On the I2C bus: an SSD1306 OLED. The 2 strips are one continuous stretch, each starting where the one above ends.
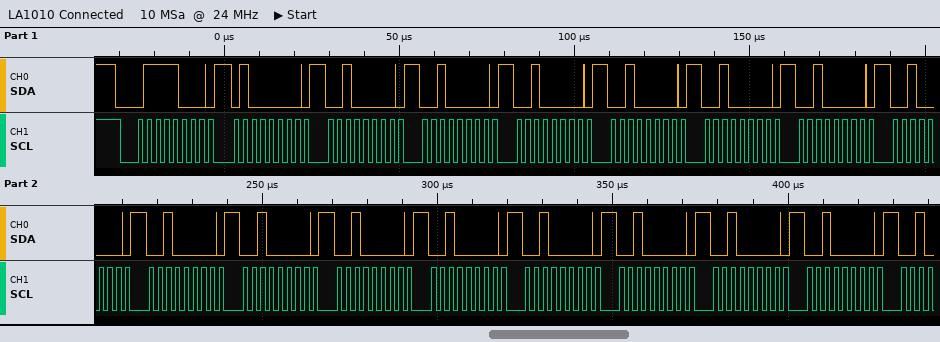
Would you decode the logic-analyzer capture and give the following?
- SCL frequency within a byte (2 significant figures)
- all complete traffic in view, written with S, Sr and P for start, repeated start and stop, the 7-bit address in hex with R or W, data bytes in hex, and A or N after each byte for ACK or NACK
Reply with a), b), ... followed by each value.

a) 400 kHz
b) S 3CW A 40 A 20 A 20 A 20 A 20 A 20 A 20 A 20 A 20 A 20 A 20 A 20 A 20 A 20 A 20 A 20 A
